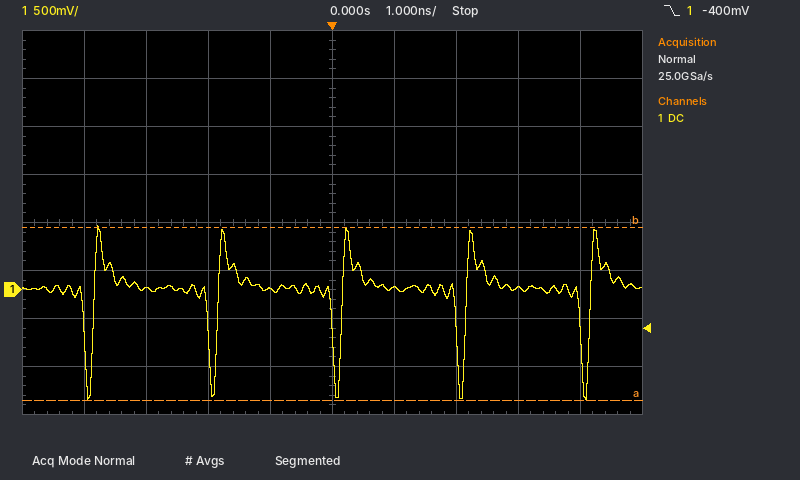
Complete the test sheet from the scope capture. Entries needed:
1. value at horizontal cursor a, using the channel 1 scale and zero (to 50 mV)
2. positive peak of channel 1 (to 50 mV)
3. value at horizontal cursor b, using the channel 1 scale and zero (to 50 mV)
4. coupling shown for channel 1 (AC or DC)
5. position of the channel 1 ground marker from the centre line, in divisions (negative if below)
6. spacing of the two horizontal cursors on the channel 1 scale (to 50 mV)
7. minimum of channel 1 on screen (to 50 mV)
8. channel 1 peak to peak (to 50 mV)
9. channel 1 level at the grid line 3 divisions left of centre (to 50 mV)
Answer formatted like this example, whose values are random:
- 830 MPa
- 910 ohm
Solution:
- -1.15 V
- 650 mV
- 650 mV
- DC
- -1.4 div
- 1.80 V
- -1.15 V
- 1.80 V
- 0 mV
